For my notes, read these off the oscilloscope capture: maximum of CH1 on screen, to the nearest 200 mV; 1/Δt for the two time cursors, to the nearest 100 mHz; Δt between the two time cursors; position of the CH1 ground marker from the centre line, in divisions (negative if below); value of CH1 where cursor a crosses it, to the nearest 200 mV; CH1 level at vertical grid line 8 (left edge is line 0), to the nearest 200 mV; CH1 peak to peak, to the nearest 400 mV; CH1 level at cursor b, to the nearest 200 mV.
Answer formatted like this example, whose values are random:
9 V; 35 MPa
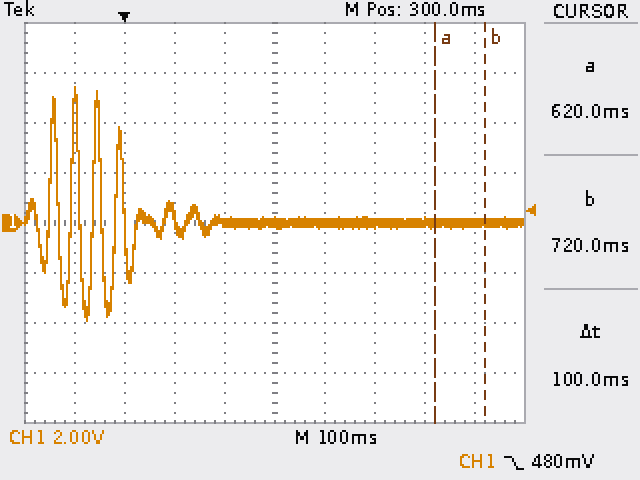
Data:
5.4 V; 10.0 Hz; 100 ms; 0.0 div; 0.0 V; 0.0 V; 9.2 V; 0.0 V
